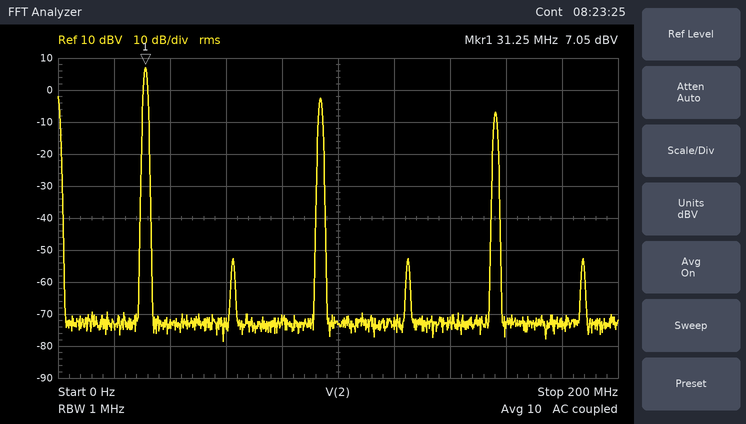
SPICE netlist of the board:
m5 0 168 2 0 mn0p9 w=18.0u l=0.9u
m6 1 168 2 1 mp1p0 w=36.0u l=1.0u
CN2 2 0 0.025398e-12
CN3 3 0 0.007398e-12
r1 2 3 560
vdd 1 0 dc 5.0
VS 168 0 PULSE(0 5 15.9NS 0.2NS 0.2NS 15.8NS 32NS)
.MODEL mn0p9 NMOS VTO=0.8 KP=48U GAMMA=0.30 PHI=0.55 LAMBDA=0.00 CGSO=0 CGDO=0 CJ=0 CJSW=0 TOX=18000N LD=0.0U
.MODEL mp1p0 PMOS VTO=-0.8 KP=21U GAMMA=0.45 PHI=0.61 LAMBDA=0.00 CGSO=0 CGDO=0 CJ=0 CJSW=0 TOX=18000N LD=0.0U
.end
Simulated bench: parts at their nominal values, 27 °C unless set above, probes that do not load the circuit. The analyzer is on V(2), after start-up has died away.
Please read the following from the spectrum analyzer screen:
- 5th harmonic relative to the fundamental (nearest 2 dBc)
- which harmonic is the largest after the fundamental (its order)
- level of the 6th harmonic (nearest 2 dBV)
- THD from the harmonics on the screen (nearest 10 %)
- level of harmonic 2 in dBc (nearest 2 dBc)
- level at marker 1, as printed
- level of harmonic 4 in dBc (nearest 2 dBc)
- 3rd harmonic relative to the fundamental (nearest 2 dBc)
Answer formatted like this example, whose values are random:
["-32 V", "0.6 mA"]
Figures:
["-14 dBc", "3", "-52 dBV", "40 %", "-60 dBc", "7.05 dBV", "-60 dBc", "-10 dBc"]
